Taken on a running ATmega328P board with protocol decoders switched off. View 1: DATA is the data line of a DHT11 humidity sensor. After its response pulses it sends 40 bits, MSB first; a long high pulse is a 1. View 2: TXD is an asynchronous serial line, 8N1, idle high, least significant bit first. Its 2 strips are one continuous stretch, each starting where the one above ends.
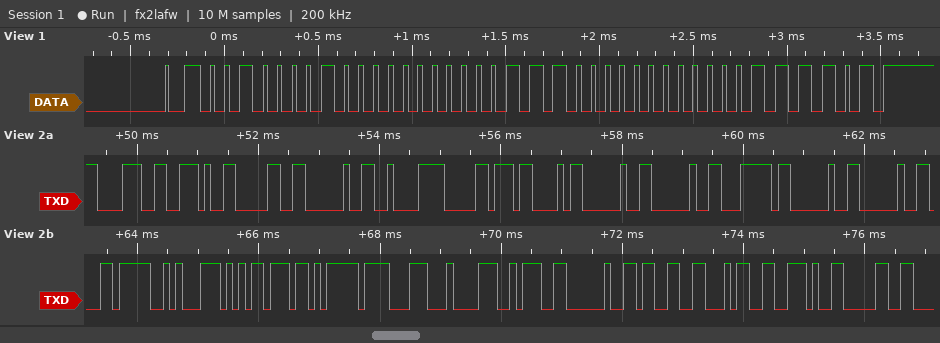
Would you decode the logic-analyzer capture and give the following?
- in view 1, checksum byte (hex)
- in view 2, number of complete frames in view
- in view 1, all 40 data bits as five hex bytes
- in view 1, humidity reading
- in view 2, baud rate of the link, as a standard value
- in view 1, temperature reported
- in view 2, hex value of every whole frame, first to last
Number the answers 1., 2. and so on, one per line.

1. 0x3D
2. 24
3. 21 00 1C 00 3D
4. 33 %
5. 9600 baud
6. 28.0 °C
7. 38 2E 30 20 C2 B0 43 20 20 7C 20 20 EC 8A B5 EB 8F 84 3A 20 33 34 2E 30
